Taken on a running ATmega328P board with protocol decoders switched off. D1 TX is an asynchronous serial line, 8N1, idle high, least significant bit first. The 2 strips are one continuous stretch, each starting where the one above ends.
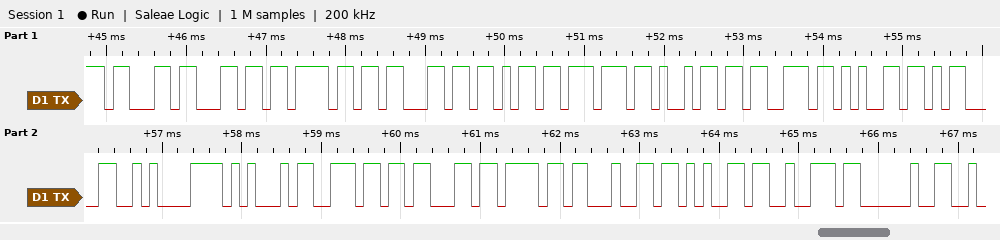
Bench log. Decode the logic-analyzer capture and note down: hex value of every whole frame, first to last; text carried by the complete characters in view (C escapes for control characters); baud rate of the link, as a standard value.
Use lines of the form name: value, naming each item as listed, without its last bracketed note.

hex value of every whole frame, first to last: 63 6C 6F 63 6B 77 69 73 65 0D 0A 45 6E 63 6F 64 65 72 20
text carried by the complete characters in view: "clockwise\r\nEncoder "
baud rate of the link, as a standard value: 9600 baud
